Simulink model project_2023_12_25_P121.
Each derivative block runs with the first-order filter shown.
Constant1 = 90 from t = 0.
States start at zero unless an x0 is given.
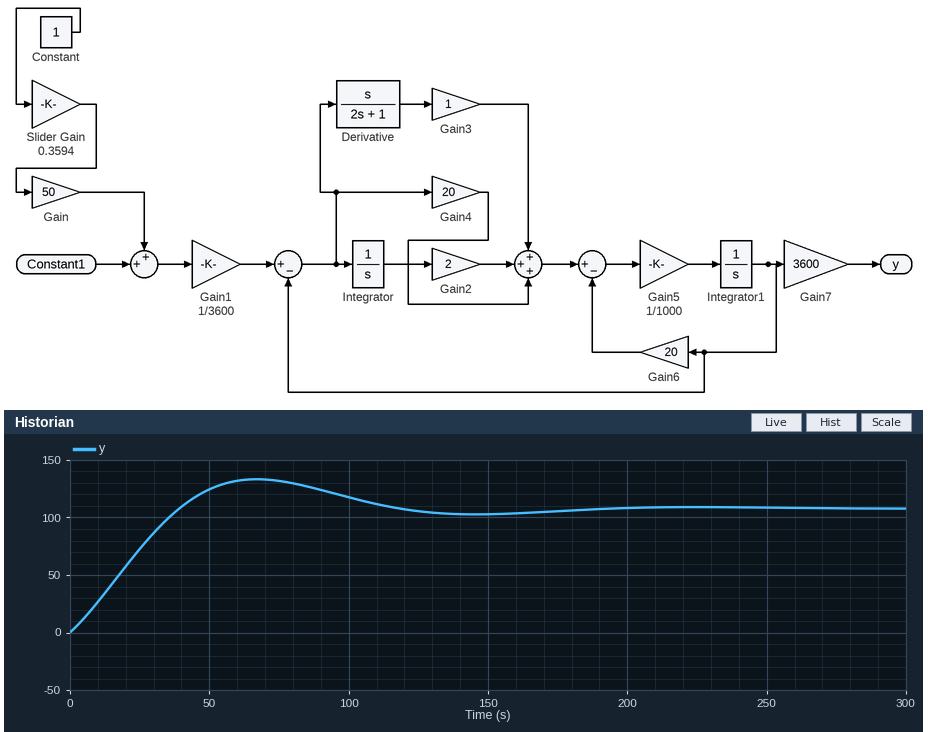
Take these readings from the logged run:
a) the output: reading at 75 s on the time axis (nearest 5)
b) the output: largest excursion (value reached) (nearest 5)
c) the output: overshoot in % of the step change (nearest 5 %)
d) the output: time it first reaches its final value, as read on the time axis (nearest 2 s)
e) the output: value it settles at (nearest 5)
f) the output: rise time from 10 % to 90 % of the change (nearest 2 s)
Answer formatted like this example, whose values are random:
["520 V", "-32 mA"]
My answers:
["130", "135", "25 %", "40 s", "110", "30 s"]
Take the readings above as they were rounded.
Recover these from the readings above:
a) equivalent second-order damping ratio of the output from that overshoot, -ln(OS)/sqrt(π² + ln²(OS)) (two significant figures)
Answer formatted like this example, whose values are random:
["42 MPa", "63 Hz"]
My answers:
["0.40"]
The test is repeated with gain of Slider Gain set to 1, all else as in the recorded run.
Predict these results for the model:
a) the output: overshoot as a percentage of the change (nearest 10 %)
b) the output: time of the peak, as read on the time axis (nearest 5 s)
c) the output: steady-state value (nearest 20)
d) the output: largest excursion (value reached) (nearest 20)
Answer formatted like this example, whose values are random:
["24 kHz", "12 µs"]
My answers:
["20 %", "65 s", "140", "180"]
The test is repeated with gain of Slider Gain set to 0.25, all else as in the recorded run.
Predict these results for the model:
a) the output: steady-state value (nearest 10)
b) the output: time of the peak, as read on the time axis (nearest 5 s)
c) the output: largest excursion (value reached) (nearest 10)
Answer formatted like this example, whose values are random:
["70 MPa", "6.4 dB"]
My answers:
["100", "65 s", "130"]
